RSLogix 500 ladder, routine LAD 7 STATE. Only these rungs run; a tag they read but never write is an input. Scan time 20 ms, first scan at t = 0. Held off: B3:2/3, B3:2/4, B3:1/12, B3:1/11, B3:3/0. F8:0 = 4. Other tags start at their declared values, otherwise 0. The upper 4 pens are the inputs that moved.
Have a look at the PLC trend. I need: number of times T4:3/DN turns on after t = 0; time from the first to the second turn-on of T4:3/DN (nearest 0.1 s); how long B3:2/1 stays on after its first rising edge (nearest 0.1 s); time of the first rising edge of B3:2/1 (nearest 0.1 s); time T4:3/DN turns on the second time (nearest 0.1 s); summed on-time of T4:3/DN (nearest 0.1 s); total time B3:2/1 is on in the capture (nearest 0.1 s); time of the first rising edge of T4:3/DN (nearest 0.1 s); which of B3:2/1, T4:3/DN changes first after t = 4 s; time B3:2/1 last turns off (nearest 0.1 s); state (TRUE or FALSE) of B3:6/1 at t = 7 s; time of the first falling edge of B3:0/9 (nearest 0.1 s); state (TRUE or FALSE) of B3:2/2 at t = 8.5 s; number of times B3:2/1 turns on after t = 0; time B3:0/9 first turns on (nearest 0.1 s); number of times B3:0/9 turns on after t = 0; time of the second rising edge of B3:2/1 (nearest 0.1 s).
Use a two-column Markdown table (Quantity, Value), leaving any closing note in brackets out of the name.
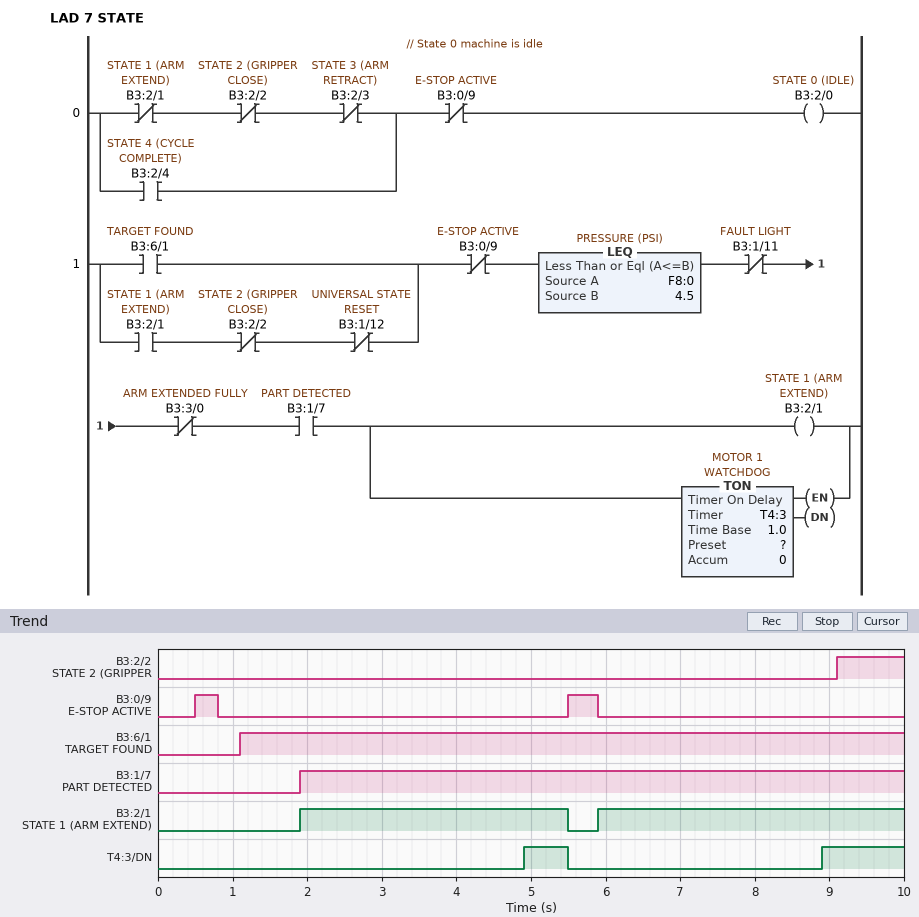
| Quantity | Value |
|---|---|
| number of times T4:3/DN turns on after t = 0 | 2 |
| time from the first to the second turn-on of T4:3/DN | 4.0 s |
| how long B3:2/1 stays on after its first rising edge | 3.6 s |
| time of the first rising edge of B3:2/1 | 1.9 s |
| time T4:3/DN turns on the second time | 8.9 s |
| summed on-time of T4:3/DN | 1.7 s |
| total time B3:2/1 is on in the capture | 7.7 s |
| time of the first rising edge of T4:3/DN | 4.9 s |
| which of B3:2/1, T4:3/DN changes first after t = 4 s | T4:3/DN |
| time B3:2/1 last turns off | 5.5 s |
| state (TRUE or FALSE) of B3:6/1 at t = 7 s | TRUE |
| time of the first falling edge of B3:0/9 | 0.8 s |
| state (TRUE or FALSE) of B3:2/2 at t = 8.5 s | FALSE |
| number of times B3:2/1 turns on after t = 0 | 2 |
| time B3:0/9 first turns on | 0.5 s |
| number of times B3:0/9 turns on after t = 0 | 2 |
| time of the second rising edge of B3:2/1 | 5.9 s |
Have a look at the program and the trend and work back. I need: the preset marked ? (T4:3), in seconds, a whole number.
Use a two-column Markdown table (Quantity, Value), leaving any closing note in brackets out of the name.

| Quantity | Value |
|---|---|
| the preset marked ? (T4:3), in seconds, a whole number | 3 s |
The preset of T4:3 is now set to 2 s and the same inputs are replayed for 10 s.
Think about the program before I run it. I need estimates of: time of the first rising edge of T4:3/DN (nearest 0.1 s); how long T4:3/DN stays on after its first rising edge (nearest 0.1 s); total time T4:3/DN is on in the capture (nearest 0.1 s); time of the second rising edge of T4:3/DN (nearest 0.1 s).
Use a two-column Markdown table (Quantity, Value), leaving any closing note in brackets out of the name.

| Quantity | Value |
|---|---|
| time of the first rising edge of T4:3/DN | 3.9 s |
| how long T4:3/DN stays on after its first rising edge | 1.6 s |
| total time T4:3/DN is on in the capture | 3.7 s |
| time of the second rising edge of T4:3/DN | 7.9 s |
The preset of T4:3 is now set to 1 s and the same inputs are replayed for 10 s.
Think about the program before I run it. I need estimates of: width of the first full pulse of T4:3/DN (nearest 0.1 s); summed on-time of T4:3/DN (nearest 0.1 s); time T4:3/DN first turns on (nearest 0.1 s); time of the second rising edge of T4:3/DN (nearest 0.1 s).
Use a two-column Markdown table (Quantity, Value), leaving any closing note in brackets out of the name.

| Quantity | Value |
|---|---|
| width of the first full pulse of T4:3/DN | 2.6 s |
| summed on-time of T4:3/DN | 5.7 s |
| time T4:3/DN first turns on | 2.9 s |
| time of the second rising edge of T4:3/DN | 6.9 s |
